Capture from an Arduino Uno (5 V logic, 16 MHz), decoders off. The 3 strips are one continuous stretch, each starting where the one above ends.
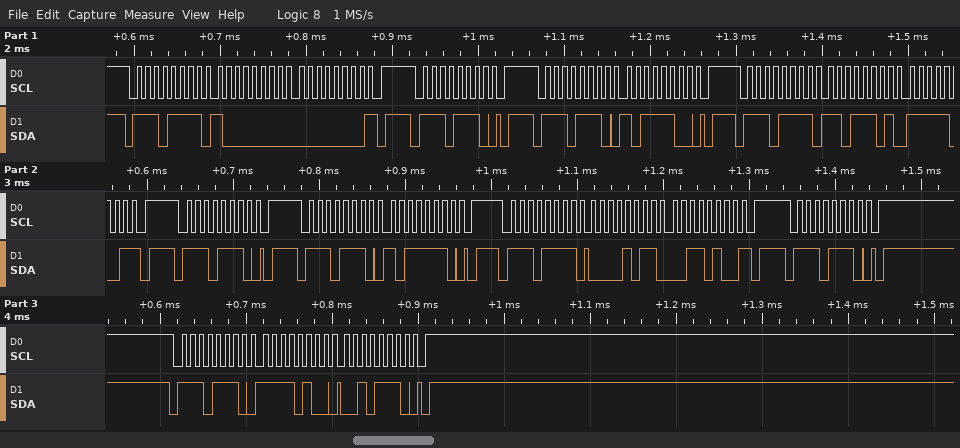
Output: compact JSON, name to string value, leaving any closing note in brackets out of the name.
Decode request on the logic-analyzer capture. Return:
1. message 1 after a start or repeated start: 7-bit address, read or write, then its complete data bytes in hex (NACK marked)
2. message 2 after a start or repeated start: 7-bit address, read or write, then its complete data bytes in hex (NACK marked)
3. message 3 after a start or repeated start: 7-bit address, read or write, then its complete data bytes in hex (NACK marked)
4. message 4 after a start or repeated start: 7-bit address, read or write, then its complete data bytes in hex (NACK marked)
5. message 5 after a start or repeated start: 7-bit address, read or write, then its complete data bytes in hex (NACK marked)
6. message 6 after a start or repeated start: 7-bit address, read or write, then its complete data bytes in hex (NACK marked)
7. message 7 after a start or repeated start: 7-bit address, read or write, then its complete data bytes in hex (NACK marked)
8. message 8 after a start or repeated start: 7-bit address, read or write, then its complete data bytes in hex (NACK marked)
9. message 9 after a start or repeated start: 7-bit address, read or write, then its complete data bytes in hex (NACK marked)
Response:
{"message 1 after a start or repeated start: 7-bit address, read or write, then its complete data bytes in hex": "0x77 read: 80 00 NACK", "message 2 after a start or repeated start: 7-bit address, read or write, then its complete data bytes in hex": "0x77 write", "message 3 after a start or repeated start: 7-bit address, read or write, then its complete data bytes in hex": "0x77 write: BC", "message 4 after a start or repeated start: 7-bit address, read or write, then its complete data bytes in hex": "0x77 read: DD F9 NACK", "message 5 after a start or repeated start: 7-bit address, read or write, then its complete data bytes in hex": "0x77 write", "message 6 after a start or repeated start: 7-bit address, read or write, then its complete data bytes in hex": "0x77 write: BE", "message 7 after a start or repeated start: 7-bit address, read or write, then its complete data bytes in hex": "0x77 read: 0B 34 NACK", "message 8 after a start or repeated start: 7-bit address, read or write, then its complete data bytes in hex": "0x77 write", "message 9 after a start or repeated start: 7-bit address, read or write, then its complete data bytes in hex": "0x77 write: F4 2E"}
